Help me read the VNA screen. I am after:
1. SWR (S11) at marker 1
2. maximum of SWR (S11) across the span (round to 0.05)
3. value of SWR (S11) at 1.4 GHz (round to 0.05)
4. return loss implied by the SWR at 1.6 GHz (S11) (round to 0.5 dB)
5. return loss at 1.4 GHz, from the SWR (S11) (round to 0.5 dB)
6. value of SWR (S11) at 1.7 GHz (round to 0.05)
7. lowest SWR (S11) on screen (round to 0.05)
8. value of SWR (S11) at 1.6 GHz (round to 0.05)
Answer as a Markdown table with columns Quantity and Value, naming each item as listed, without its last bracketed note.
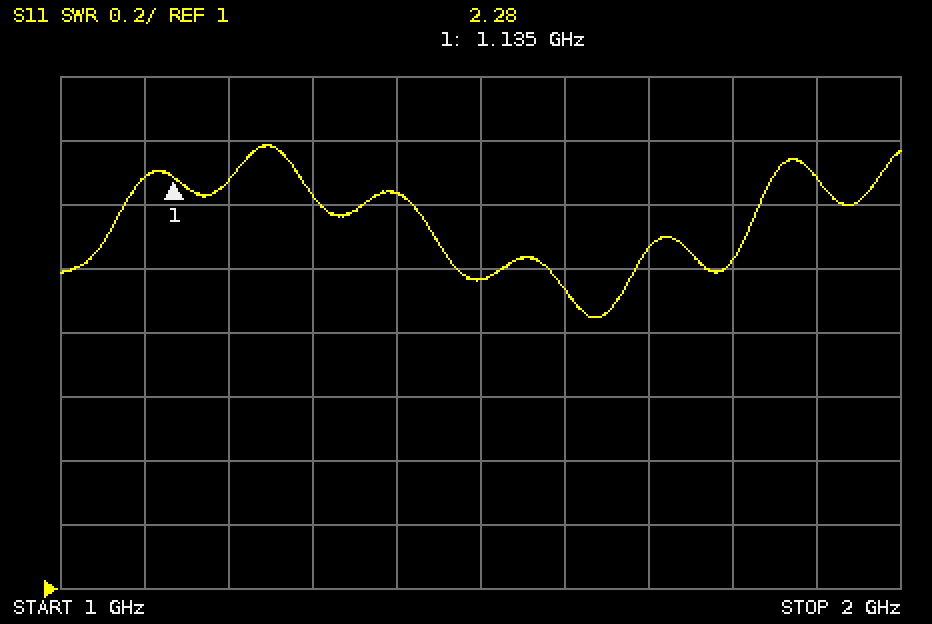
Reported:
| Quantity | Value |
|---|---|
| SWR (S11) at marker 1 | 2.28 |
| maximum of SWR (S11) across the span | 2.40 |
| value of SWR (S11) at 1.4 GHz | 2.25 |
| return loss implied by the SWR at 1.6 GHz (S11) | 10.0 dB |
| return loss at 1.4 GHz, from the SWR (S11) | 8.5 dB |
| value of SWR (S11) at 1.7 GHz | 2.05 |
| lowest SWR (S11) on screen | 1.85 |
| value of SWR (S11) at 1.6 GHz | 1.95 |
